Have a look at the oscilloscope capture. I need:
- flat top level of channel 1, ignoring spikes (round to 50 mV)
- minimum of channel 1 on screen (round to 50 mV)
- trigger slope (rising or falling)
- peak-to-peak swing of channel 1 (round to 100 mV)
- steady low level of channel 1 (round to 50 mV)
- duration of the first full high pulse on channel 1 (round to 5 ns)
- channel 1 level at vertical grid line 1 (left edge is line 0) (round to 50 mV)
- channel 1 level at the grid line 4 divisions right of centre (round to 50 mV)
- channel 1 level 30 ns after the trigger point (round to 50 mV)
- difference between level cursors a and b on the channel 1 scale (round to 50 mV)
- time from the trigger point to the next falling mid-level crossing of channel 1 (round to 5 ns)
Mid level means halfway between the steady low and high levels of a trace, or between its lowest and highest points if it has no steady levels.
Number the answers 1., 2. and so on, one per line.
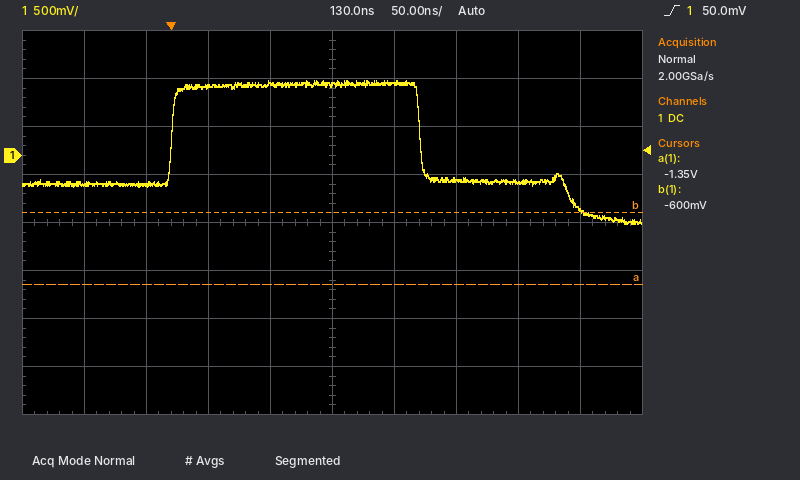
1. 750 mV
2. -700 mV
3. rising
4. 1.50 V
5. -300 mV
6. 200 ns
7. -300 mV
8. -550 mV
9. 700 mV
10. 750 mV
11. 200 ns
